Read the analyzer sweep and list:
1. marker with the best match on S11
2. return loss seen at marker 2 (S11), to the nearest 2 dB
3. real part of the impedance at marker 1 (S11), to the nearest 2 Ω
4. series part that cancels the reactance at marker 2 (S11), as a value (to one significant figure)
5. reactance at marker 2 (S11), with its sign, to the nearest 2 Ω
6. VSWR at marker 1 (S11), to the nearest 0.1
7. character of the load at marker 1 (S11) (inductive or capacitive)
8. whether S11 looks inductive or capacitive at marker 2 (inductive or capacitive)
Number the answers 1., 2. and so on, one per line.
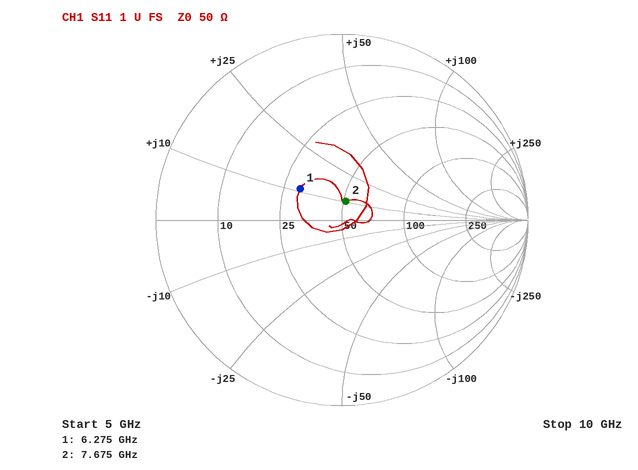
1. marker 2
2. 20 dB
3. 30 Ω
4. 2 pF
5. +10 Ω
6. 1.8
7. inductive
8. inductive
